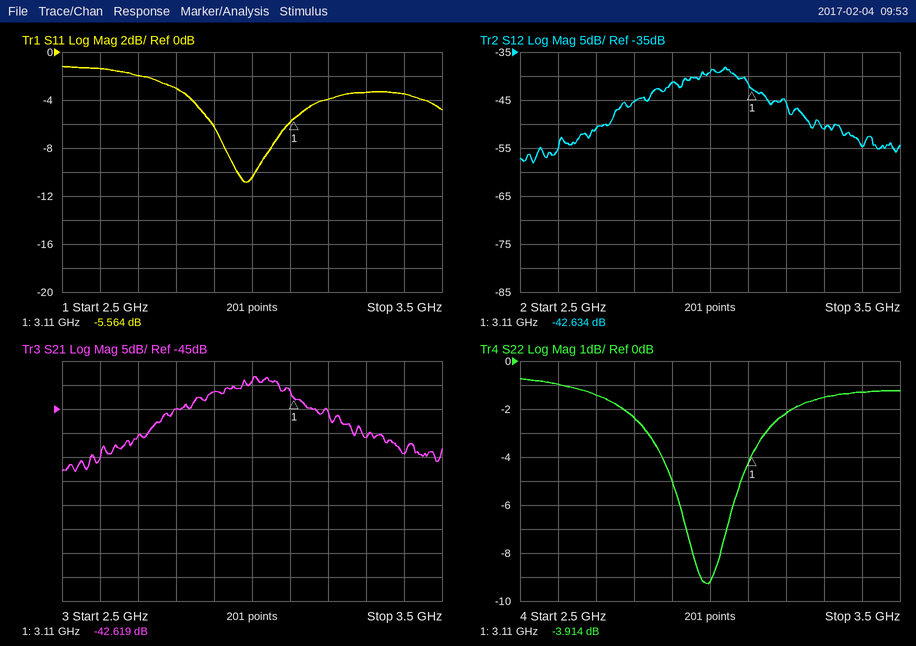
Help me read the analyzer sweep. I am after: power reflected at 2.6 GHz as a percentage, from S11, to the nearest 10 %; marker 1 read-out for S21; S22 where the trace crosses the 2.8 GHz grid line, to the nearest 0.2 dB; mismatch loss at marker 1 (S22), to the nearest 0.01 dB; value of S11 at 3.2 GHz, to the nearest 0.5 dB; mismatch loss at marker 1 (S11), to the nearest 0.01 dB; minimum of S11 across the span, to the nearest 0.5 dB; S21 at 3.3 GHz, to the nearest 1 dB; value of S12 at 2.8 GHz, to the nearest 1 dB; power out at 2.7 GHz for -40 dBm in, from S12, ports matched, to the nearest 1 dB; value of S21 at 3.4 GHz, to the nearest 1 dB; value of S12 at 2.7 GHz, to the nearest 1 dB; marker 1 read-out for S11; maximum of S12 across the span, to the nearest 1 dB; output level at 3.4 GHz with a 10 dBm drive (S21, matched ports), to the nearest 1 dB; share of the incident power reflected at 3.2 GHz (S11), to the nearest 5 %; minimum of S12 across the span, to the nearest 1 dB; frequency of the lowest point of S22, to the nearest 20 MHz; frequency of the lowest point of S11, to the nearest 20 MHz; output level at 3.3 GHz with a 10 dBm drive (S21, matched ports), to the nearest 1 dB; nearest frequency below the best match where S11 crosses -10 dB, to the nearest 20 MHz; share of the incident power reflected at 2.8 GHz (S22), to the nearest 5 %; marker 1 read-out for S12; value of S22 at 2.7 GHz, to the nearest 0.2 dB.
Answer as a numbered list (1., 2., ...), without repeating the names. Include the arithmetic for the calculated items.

1. 10^(-1.5/10) ≈ 70.8 %, so 70 % to the nearest 10 %
2. -42.619 dB
3. -2.4 dB
4. −10 log10(1 − 10^(-3.914/10)) ≈ 2.26 dB
5. -4.0 dB
6. −10 log10(1 − 10^(-5.564/10)) ≈ 1.41 dB
7. -11.0 dB
8. -51 dB
9. -45 dB
10. -40 dBm + (-51 dB) = -91 dBm
11. -54 dB
12. -51 dB
13. -5.564 dB
14. -38 dB
15. 10 dBm + (-54 dB) = -44 dBm
16. 10^(-4/10) ≈ 40 %
17. -58 dB
18. 3.00 GHz
19. 2.98 GHz
20. 10 dBm + (-51 dB) = -41 dBm
21. 2.96 GHz
22. 10^(-2.4/10) ≈ 57.5 %, so 60 % to the nearest 5 %
23. -42.634 dB
24. -1.4 dB
